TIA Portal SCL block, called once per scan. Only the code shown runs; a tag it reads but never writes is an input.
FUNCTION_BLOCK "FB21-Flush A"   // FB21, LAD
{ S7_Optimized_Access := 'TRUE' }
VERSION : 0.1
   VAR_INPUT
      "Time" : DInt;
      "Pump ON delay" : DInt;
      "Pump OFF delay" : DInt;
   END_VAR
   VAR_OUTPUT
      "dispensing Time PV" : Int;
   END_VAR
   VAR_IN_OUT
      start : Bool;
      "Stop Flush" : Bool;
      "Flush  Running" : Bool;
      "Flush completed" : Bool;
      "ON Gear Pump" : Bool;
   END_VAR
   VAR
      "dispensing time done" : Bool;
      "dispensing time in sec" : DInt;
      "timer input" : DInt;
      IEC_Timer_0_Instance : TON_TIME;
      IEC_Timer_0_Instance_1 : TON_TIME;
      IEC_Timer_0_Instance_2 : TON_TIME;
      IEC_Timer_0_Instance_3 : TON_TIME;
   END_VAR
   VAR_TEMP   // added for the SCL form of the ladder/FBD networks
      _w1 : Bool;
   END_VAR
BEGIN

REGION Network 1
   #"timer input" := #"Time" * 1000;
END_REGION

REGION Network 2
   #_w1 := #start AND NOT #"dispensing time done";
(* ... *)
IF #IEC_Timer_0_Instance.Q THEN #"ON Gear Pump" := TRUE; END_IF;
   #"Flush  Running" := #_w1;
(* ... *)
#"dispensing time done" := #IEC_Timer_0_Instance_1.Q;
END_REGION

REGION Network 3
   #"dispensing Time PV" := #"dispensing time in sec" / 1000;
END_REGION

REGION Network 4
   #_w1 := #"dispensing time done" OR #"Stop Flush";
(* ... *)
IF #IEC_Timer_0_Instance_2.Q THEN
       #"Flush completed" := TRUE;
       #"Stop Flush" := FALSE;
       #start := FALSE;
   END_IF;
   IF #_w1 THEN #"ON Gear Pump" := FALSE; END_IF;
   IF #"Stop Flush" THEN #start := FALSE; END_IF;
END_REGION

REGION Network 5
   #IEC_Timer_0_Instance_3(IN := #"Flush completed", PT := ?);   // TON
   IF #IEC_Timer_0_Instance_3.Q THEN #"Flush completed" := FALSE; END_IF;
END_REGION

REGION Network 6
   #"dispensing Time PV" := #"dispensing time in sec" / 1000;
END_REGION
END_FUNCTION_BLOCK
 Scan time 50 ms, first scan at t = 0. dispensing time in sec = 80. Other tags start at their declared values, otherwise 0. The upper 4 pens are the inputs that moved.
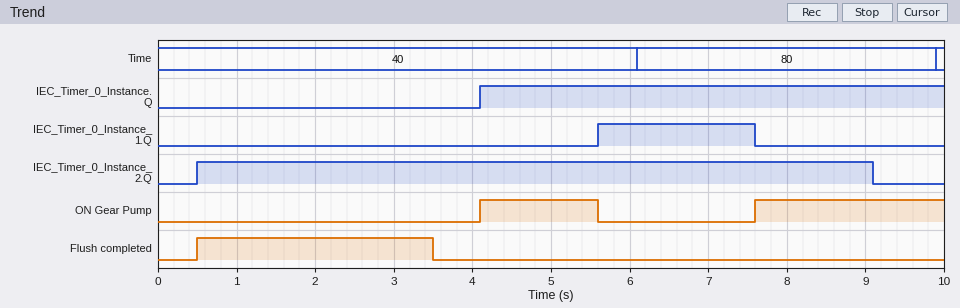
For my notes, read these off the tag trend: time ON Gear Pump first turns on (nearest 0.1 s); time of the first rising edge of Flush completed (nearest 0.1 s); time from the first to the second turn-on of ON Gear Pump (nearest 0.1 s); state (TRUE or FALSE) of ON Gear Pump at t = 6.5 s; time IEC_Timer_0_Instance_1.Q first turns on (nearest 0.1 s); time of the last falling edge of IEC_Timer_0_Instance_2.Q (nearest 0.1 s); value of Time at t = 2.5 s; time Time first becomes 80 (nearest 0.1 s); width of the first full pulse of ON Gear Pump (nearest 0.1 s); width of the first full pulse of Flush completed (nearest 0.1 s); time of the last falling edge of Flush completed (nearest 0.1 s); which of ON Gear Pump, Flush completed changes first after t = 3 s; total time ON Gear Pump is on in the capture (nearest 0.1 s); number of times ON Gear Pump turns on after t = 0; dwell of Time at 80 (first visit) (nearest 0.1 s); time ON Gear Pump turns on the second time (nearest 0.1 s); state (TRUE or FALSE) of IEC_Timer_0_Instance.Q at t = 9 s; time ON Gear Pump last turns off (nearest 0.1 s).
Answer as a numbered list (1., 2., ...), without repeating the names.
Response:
1. 4.1 s
2. 0.5 s
3. 3.5 s
4. FALSE
5. 5.6 s
6. 9.1 s
7. 40
8. 6.1 s
9. 1.5 s
10. 3.0 s
11. 3.5 s
12. Flush completed
13. 3.9 s
14. 2
15. 3.8 s
16. 7.6 s
17. TRUE
18. 5.6 s
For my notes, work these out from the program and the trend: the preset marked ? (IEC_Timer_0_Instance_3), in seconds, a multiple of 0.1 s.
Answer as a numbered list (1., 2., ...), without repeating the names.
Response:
1. 3.0 s
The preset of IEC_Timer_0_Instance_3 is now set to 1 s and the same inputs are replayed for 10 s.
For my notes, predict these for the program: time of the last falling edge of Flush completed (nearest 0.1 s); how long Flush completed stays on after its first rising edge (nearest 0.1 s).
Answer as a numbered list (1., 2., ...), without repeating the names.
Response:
1. 1.5 s
2. 1.0 s
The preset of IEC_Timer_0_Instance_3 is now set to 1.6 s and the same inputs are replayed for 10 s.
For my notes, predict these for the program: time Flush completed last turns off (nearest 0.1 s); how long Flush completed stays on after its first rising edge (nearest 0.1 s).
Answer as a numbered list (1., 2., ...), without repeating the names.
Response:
1. 2.1 s
2. 1.6 s
